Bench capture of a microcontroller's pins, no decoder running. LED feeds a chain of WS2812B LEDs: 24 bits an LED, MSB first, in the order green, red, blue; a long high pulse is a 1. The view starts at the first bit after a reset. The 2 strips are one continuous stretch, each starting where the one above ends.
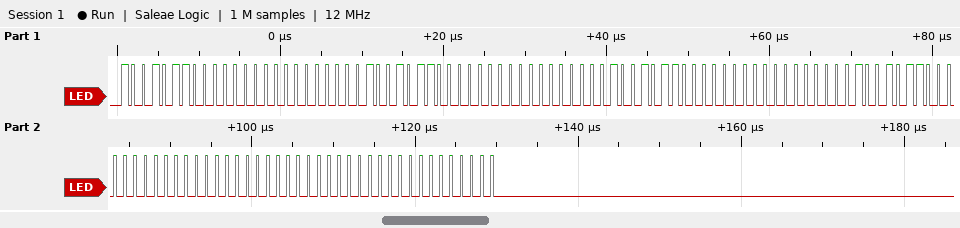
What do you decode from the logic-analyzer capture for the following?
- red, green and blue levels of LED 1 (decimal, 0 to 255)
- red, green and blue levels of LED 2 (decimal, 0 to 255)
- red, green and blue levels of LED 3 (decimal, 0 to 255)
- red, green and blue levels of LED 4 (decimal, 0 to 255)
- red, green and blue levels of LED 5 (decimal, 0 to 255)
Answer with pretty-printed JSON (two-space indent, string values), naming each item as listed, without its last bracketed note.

{
  "red, green and blue levels of LED 1": "0, 150, 0",
  "red, green and blue levels of LED 2": "0, 150, 0",
  "red, green and blue levels of LED 3": "0, 150, 0",
  "red, green and blue levels of LED 4": "0, 150, 0",
  "red, green and blue levels of LED 5": "0, 0, 0"
}
